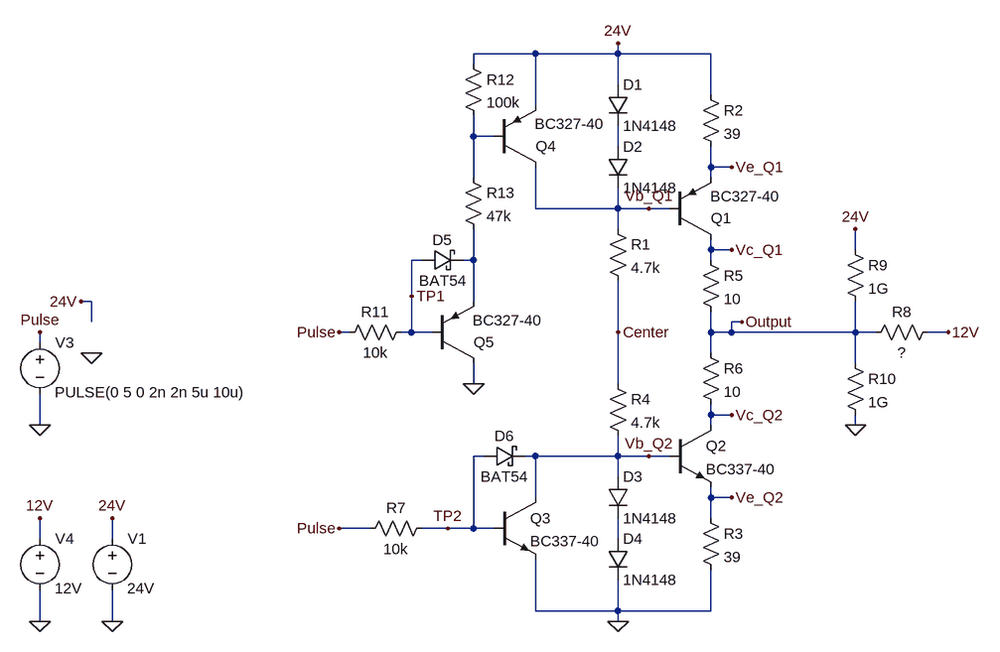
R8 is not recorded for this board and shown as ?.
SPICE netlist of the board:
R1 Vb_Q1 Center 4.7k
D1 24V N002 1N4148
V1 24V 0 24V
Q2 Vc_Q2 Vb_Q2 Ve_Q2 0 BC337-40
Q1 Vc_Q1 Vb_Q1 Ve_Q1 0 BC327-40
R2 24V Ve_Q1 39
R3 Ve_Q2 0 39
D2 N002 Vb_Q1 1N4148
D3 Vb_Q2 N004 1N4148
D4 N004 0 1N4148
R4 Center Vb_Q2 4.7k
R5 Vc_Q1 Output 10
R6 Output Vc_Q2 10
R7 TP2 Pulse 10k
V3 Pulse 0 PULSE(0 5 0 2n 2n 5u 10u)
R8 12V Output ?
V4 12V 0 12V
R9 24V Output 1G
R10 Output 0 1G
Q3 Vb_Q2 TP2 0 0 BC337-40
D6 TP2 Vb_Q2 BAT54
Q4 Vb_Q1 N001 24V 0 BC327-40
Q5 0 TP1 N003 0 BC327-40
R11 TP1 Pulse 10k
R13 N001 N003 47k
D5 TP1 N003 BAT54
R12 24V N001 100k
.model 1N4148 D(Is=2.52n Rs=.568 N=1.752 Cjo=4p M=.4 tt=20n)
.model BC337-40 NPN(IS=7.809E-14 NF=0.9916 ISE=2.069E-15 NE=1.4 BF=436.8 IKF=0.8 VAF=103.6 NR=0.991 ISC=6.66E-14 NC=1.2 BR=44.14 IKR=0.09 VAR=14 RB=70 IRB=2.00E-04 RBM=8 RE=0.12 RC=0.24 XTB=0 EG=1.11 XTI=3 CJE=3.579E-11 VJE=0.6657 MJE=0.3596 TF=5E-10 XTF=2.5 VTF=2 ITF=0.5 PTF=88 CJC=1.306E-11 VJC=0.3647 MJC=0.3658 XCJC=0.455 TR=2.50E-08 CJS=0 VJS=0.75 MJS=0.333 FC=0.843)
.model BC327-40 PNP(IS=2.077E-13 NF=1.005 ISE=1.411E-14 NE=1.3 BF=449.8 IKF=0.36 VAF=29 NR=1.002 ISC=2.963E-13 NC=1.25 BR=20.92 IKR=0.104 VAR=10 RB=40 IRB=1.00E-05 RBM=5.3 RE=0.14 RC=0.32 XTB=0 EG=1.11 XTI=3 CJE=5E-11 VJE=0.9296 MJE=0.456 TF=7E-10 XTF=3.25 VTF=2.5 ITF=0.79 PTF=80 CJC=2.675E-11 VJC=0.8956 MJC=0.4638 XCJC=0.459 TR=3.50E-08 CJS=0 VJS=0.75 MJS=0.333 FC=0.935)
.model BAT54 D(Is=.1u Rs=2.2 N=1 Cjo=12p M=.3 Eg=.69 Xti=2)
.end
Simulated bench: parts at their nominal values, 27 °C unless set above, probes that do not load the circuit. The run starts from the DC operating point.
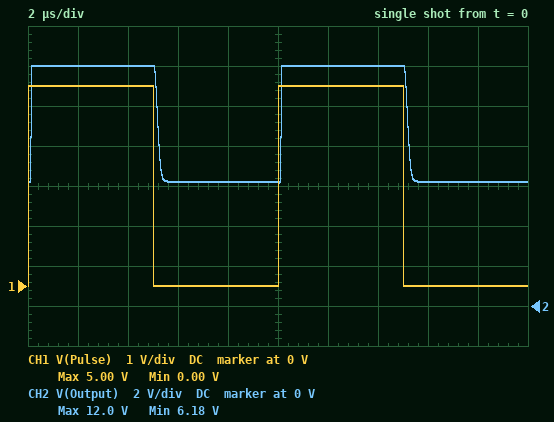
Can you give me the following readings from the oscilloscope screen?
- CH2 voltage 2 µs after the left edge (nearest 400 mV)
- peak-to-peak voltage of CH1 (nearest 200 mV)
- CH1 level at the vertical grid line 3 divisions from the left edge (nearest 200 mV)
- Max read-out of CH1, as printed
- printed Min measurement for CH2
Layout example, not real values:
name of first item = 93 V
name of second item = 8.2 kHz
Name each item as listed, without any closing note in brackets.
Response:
CH2 voltage 2 µs after the left edge = 12.0 V
peak-to-peak voltage of CH1 = 5.0 V
CH1 level at the vertical grid line 3 divisions from the left edge = 0 V
Max read-out of CH1, as printed = 5.00 V
printed Min measurement for CH2 = 6.18 V
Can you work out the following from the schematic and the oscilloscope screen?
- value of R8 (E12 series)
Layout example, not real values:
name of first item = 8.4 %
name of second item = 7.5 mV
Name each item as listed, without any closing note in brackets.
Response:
value of R8 = 390 Ω
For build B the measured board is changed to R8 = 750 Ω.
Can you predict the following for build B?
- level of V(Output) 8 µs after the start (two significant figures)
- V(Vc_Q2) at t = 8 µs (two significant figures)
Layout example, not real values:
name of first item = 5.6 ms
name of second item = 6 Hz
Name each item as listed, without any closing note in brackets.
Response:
level of V(Output) 8 µs after the start = 910 mV
V(Vc_Q2) at t = 8 µs = 770 mV
